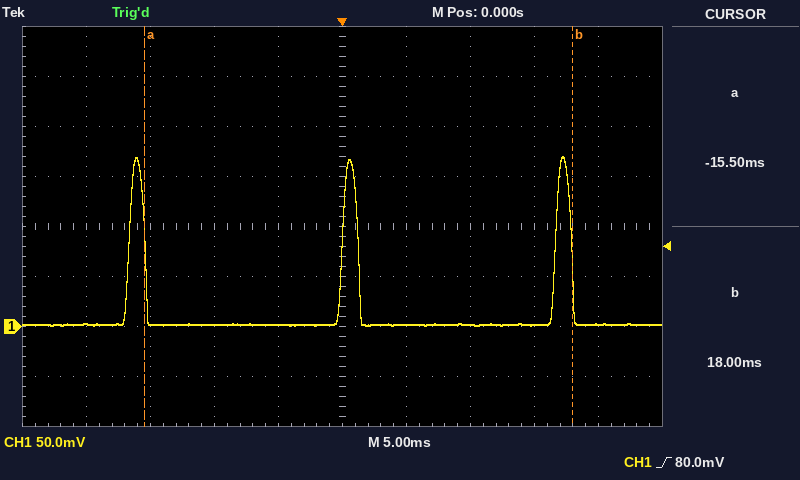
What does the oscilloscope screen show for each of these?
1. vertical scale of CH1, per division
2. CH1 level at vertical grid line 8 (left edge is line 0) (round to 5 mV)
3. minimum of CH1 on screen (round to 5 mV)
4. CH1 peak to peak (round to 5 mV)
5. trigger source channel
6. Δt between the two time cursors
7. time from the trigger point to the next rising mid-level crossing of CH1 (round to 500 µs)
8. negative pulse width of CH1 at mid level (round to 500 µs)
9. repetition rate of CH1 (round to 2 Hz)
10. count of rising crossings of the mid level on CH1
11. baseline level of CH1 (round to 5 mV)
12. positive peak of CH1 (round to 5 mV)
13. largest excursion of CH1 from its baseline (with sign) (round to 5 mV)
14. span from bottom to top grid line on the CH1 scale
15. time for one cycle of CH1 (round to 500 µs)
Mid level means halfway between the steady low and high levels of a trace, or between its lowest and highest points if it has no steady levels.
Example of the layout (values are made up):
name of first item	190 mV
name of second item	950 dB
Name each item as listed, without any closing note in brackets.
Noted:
vertical scale of CH1, per division	50 mV
CH1 level at vertical grid line 8 (left edge is line 0)	0 mV
minimum of CH1 on screen	0 mV
CH1 peak to peak	170 mV
trigger source channel	CH1
Δt between the two time cursors	33.5 ms
time from the trigger point to the next rising mid-level crossing of CH1	16.5 ms
negative pulse width of CH1 at mid level	15.5 ms
repetition rate of CH1	60 Hz
count of rising crossings of the mid level on CH1	3
baseline level of CH1	0 mV
positive peak of CH1	170 mV
largest excursion of CH1 from its baseline (with sign)	+170 mV
span from bottom to top grid line on the CH1 scale	400 mV
time for one cycle of CH1	16.5 ms
